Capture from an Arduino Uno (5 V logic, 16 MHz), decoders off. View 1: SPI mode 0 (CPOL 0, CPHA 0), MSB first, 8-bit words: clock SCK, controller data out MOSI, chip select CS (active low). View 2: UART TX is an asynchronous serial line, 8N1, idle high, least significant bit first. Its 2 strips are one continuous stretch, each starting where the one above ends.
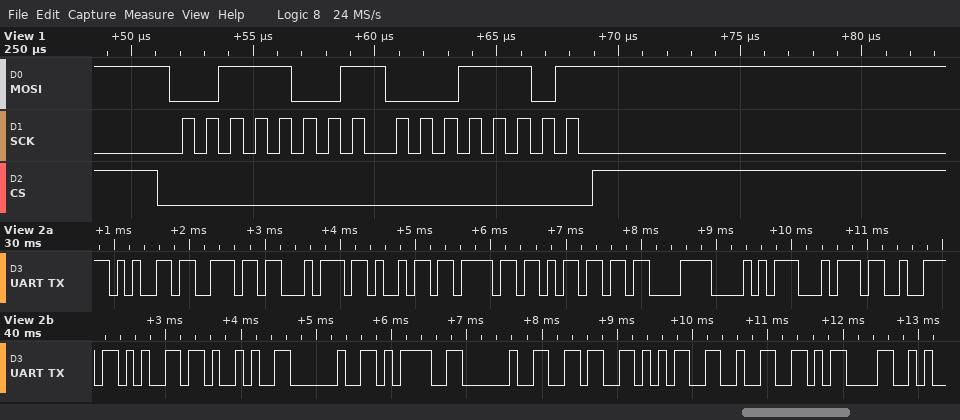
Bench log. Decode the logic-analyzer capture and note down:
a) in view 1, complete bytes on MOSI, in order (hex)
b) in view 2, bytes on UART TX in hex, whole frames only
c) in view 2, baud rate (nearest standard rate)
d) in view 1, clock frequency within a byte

39 1D
0x65 0x6E 0x74 0x69 0x6F 0x6D 0xC3 0xA8 0x74 0x72 0x65 0x29 0x20 0x3D 0x20 0x36 0x35 0x32 0x0D
9600 baud
1 MHz
